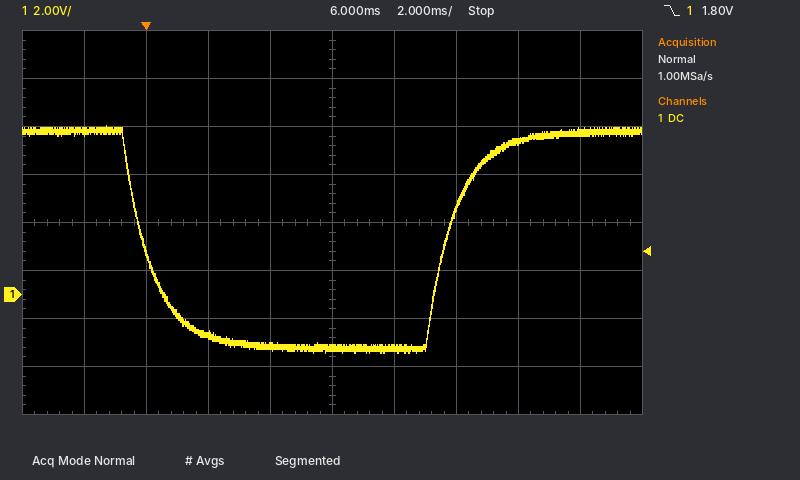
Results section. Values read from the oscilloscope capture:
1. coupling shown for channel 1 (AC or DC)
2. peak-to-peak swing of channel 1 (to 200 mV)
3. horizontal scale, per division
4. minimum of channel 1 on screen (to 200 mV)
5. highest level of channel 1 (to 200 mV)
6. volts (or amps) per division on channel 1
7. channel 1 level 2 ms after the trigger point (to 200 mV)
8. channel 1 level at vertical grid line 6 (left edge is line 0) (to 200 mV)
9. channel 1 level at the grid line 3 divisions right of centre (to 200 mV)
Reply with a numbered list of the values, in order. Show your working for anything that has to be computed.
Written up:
1. DC
2. 7.0 V − (-2.4 V) = 9.4 V
3. 2 ms
4. -2.4 V
5. 7.0 V
6. 2 V
7. -1.6 V
8. -2.2 V
9. 6.4 V
